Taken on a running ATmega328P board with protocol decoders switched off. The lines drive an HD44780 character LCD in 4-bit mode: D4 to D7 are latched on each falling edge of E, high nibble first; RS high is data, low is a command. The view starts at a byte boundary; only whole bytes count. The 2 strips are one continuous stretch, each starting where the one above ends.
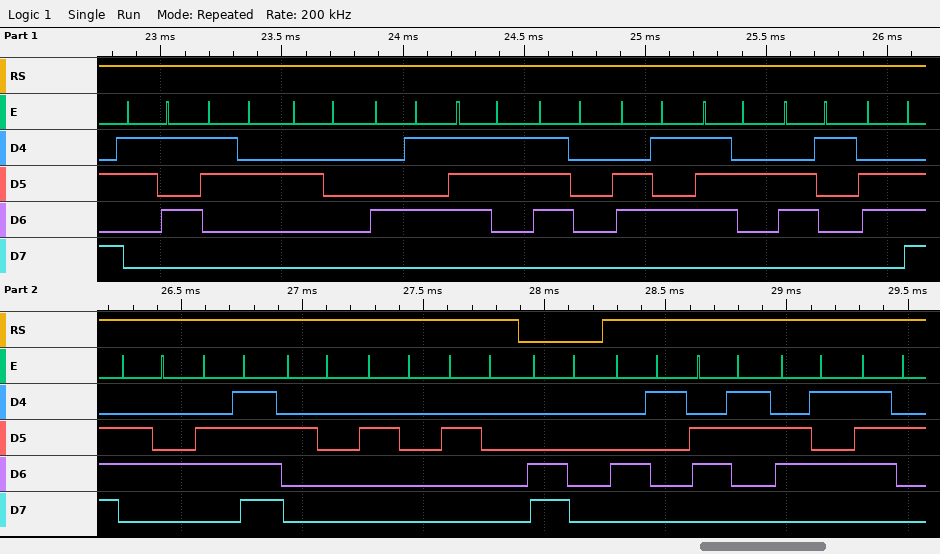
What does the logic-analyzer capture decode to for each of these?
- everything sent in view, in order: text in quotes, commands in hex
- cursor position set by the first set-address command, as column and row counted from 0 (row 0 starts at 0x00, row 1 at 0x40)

"52 Esperando   " 0xC0 "Acer"
column 0, row 1
